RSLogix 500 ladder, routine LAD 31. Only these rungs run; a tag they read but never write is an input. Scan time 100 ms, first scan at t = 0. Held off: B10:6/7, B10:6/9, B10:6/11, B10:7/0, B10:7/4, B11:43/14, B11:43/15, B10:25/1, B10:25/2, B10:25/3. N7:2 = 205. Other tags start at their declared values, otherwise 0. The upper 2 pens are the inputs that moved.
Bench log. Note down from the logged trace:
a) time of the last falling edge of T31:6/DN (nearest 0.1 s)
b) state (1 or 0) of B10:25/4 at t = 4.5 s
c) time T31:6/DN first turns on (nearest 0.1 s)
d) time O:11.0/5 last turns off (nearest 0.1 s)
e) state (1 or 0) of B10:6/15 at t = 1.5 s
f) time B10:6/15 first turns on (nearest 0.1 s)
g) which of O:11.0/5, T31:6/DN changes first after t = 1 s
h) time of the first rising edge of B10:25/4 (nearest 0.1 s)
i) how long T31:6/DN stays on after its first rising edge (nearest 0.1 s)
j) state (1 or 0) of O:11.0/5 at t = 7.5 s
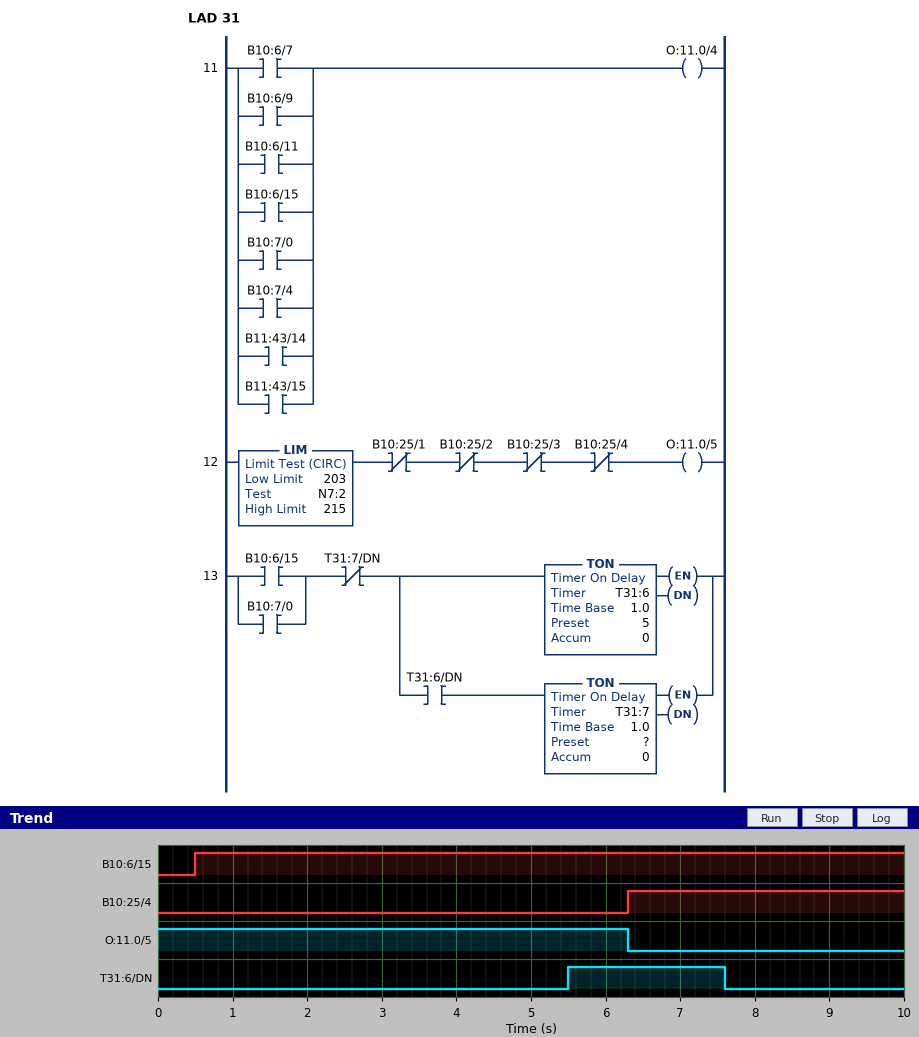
7.6 s
0
5.5 s
6.3 s
1
0.5 s
T31:6/DN
6.3 s
2.1 s
0
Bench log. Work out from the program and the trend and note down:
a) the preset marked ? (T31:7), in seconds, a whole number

2 s
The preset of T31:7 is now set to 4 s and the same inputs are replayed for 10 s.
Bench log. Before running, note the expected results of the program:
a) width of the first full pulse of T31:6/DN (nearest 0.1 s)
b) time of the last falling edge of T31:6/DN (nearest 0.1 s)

4.1 s
9.6 s
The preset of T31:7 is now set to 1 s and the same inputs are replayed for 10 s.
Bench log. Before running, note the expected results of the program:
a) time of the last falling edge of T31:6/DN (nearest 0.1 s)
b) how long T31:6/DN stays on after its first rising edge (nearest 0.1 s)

6.6 s
1.1 s
